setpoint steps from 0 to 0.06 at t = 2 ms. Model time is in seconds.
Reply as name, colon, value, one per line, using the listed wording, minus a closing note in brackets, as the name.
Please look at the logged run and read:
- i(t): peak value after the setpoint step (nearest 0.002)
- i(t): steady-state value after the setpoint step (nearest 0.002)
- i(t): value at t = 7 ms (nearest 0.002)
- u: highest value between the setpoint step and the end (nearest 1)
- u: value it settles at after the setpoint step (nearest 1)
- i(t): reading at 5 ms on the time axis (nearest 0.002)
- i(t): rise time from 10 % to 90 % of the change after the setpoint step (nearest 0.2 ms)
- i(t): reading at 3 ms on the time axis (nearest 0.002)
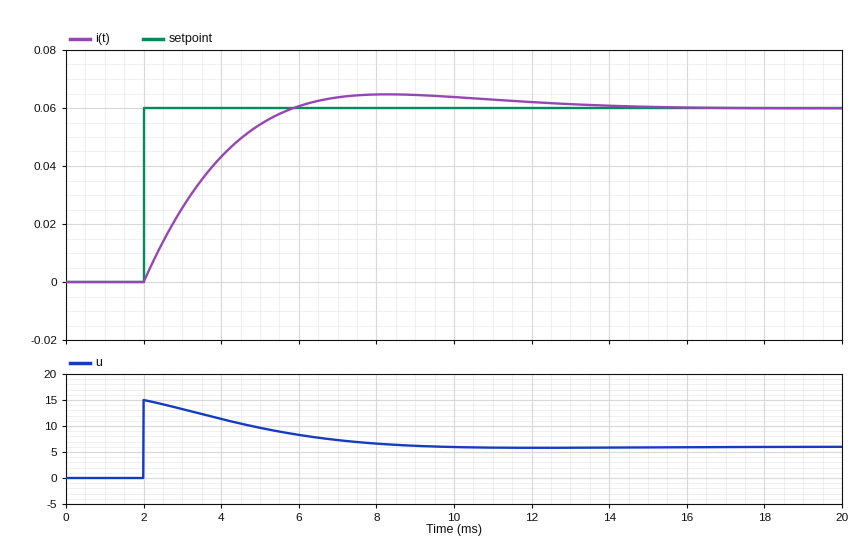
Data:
i(t): peak value after the setpoint step: 0.064
i(t): steady-state value after the setpoint step: 0.060
i(t): value at t = 7 ms: 0.064
u: highest value between the setpoint step and the end: 15
u: value it settles at after the setpoint step: 6
i(t): reading at 5 ms on the time axis: 0.054
i(t): rise time from 10 % to 90 % of the change after the setpoint step: 2.8 ms
i(t): reading at 3 ms on the time axis: 0.026
